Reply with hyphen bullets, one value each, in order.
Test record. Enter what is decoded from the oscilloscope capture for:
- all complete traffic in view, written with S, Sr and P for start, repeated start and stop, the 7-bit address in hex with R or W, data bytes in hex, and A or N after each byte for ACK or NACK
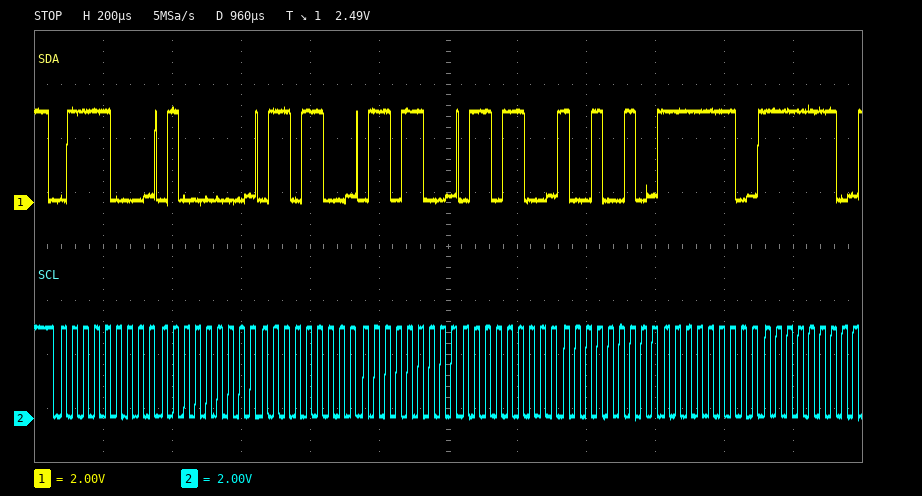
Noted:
- S 3CW A 40 A 6C A 6C A 6C A 92 A FE A FE A
